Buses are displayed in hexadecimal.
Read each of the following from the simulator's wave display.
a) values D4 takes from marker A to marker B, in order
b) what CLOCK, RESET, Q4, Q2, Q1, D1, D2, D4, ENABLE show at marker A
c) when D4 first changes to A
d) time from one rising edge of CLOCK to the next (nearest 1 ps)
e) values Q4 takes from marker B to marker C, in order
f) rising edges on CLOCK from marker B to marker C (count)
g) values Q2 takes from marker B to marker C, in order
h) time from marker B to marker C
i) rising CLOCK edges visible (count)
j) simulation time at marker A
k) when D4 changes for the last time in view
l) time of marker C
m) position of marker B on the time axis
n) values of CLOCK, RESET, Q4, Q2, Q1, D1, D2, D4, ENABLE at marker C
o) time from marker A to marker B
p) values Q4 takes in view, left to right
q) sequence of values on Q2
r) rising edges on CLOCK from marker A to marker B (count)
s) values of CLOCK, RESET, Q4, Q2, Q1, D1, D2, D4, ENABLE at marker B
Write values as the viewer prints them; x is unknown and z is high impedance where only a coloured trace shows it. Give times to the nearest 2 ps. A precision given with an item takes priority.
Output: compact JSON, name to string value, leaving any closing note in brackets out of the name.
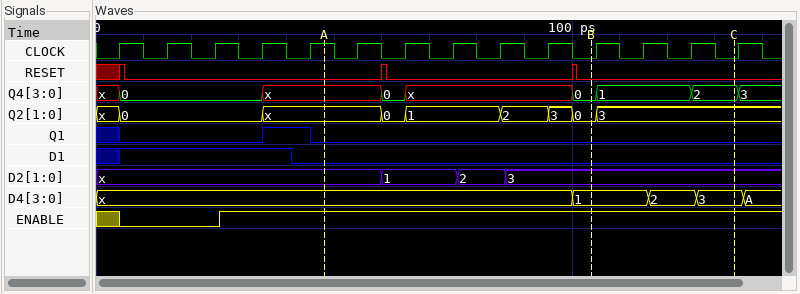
{"values D4 takes from marker A to marker B, in order": "x, 1", "what CLOCK, RESET, Q4, Q2, Q1, D1, D2, D4, ENABLE show at marker A": "CLOCK=1, RESET=0, Q4=x, Q2=x, Q1=0, D1=0, D2=x, D4=x, ENABLE=1", "when D4 first changes to A": "136 ps", "time from one rising edge of CLOCK to the next": "10 ps", "values Q4 takes from marker B to marker C, in order": "0, 1, 2", "rising edges on CLOCK from marker B to marker C": "3", "values Q2 takes from marker B to marker C, in order": "0, 3", "time from marker B to marker C": "30 ps", "rising CLOCK edges visible": "14", "simulation time at marker A": "48 ps", "when D4 changes for the last time in view": "136 ps", "time of marker C": "134 ps", "position of marker B on the time axis": "104 ps", "values of CLOCK, RESET, Q4, Q2, Q1, D1, D2, D4, ENABLE at marker C": "CLOCK=0, RESET=0, Q4=2, Q2=3, Q1=0, D1=0, D2=3, D4=3, ENABLE=1", "time from marker A to marker B": "56 ps", "values Q4 takes in view, left to right": "x, 0, x, 0, x, 0, 1, 2, 3", "sequence of values on Q2": "x, 0, x, 0, 1, 2, 3, 0, 3", "rising edges on CLOCK from marker A to marker B": "5", "values of CLOCK, RESET, Q4, Q2, Q1, D1, D2, D4, ENABLE at marker B": "CLOCK=0, RESET=0, Q4=0, Q2=0, Q1=0, D1=0, D2=3, D4=1, ENABLE=1"}
